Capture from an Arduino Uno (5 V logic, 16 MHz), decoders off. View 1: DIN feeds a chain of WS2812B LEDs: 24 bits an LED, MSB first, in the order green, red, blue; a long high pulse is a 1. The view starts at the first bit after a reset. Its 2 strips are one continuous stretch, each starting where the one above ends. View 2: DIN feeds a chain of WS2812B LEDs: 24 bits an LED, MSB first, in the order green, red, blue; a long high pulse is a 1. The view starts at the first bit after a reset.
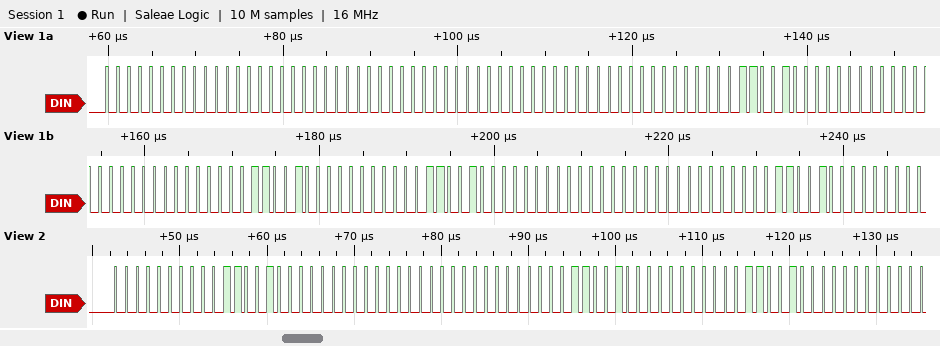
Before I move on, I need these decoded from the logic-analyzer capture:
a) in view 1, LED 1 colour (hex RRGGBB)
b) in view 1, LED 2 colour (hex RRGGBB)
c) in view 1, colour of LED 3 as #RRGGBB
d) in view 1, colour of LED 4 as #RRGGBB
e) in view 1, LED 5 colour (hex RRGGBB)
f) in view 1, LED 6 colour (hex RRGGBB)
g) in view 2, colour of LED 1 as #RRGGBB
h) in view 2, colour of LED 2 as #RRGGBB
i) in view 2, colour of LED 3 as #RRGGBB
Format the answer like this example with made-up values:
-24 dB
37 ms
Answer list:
#000000
#000000
#320000
#000032
#320000
#000032
#320000
#000032
#320000
